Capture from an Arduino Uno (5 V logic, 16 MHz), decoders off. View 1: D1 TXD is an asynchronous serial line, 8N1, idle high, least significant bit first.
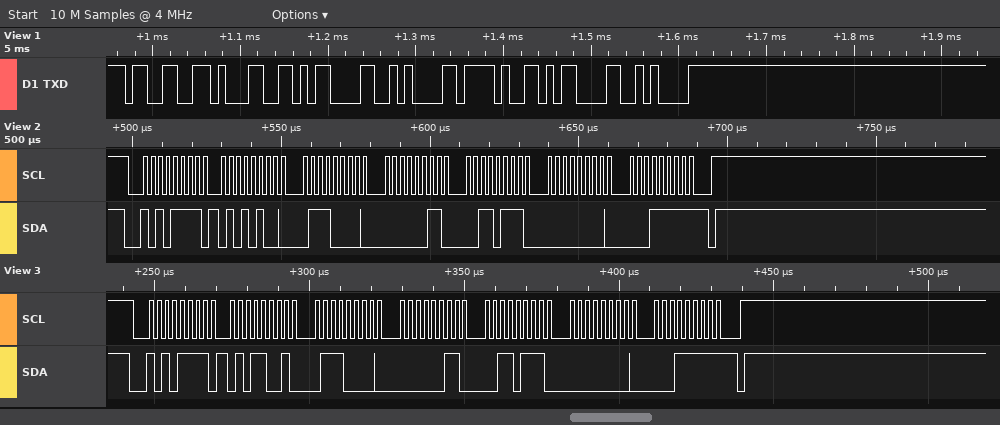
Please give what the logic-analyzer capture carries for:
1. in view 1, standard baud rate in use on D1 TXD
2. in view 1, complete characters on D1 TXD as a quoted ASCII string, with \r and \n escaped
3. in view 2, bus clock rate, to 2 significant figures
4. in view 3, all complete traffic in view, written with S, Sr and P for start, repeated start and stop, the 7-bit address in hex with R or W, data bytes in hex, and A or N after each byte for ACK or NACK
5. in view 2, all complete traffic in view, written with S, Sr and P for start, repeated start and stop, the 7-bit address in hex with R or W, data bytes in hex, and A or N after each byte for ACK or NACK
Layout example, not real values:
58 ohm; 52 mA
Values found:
115200 baud; "31\r\n/\r\n"; 400 kHz; S 57R A 59 A 70 A 03 A 37 A 00 A 1F N P; S 57R A 54 A 70 A 03 A 37 A 00 A 1F N P
